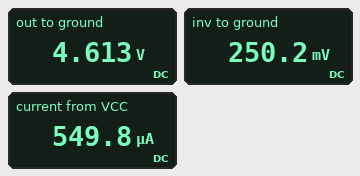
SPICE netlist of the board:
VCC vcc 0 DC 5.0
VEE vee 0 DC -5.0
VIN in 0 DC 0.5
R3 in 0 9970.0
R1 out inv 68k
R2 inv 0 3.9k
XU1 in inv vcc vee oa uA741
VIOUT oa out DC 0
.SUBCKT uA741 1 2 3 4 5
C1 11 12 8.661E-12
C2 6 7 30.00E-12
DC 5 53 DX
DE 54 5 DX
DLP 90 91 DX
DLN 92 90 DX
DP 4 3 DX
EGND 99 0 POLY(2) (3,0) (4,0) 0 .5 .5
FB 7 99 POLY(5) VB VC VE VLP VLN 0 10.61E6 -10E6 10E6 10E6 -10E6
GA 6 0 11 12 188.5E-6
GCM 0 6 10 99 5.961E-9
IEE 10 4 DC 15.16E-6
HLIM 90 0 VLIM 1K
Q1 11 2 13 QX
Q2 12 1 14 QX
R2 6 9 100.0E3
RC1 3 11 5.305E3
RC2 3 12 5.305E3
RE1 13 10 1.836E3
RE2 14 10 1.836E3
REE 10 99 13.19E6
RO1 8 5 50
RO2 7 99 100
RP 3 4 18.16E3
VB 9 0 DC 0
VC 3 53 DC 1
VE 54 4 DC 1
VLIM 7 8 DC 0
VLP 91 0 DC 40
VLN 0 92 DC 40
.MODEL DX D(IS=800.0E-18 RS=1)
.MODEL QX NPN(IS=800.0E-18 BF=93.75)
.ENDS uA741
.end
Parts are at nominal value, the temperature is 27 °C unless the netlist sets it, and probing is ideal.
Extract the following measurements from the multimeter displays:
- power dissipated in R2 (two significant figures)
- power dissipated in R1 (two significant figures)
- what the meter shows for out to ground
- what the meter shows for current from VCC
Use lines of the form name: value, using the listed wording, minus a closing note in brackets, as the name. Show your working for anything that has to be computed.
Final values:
power dissipated in R2: (250.2 mV)^2 / 3.9 kΩ = 16 µW
power dissipated in R1: (4.613 V - 250.2 mV)^2 / 68 kΩ = 280 µW
what the meter shows for out to ground: 4.613 V
what the meter shows for current from VCC: 549.8 µA
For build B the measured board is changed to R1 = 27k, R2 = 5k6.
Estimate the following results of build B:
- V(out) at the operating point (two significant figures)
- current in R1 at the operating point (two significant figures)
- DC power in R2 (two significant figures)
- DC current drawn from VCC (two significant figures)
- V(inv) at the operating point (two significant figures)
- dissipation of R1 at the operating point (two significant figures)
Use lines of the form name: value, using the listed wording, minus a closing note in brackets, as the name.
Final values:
V(out) at the operating point: 2.9 V
current in R1 at the operating point: 89 µA
DC power in R2: 45 µW
DC current drawn from VCC: 570 µA
V(inv) at the operating point: 500 mV
dissipation of R1 at the operating point: 220 µW
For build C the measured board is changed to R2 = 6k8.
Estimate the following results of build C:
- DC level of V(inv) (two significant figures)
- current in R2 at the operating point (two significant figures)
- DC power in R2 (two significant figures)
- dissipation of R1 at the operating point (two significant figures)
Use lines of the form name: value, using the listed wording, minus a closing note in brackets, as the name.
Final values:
DC level of V(inv): 420 mV
current in R2 at the operating point: 62 µA
DC power in R2: 26 µW
dissipation of R1 at the operating point: 260 µW
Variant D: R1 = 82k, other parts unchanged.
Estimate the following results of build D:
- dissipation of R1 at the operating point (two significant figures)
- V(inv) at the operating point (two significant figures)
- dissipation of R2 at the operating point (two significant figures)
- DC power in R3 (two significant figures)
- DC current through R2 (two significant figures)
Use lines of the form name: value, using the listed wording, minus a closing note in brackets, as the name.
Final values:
dissipation of R1 at the operating point: 240 µW
V(inv) at the operating point: 210 mV
dissipation of R2 at the operating point: 11 µW
DC power in R3: 25 µW
DC current through R2: 54 µA
